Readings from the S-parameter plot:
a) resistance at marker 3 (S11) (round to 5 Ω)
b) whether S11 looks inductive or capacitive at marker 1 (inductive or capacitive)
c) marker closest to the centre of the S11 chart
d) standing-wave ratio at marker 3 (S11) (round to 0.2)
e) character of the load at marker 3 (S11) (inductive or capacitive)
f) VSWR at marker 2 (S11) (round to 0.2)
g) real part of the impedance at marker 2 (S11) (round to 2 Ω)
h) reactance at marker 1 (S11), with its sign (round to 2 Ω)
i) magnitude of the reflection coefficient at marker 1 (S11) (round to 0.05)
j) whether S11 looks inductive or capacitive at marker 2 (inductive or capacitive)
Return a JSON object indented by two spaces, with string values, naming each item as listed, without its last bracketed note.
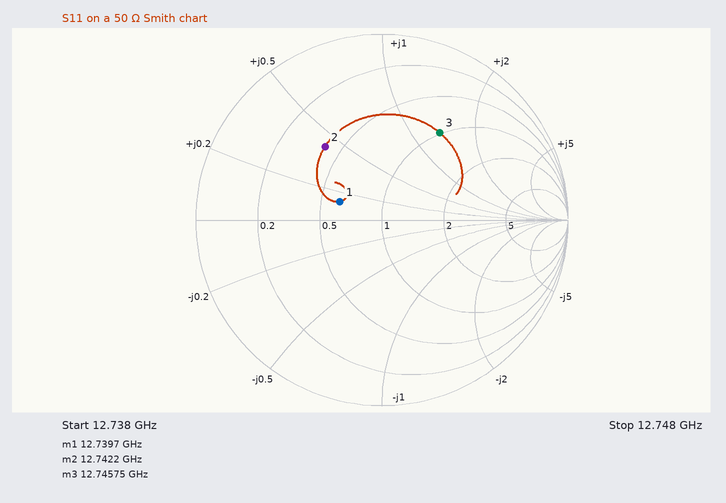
{
  "resistance at marker 3 (S11)": "50 Ω",
  "whether S11 looks inductive or capacitive at marker 1": "inductive",
  "marker closest to the centre of the S11 chart": "marker 1",
  "standing-wave ratio at marker 3 (S11)": "3.6",
  "character of the load at marker 3 (S11)": "inductive",
  "VSWR at marker 2 (S11)": "3.0",
  "real part of the impedance at marker 2 (S11)": "20 Ω",
  "reactance at marker 1 (S11), with its sign": "+6 Ω",
  "magnitude of the reflection coefficient at marker 1 (S11)": "0.25",
  "whether S11 looks inductive or capacitive at marker 2": "inductive"
}
